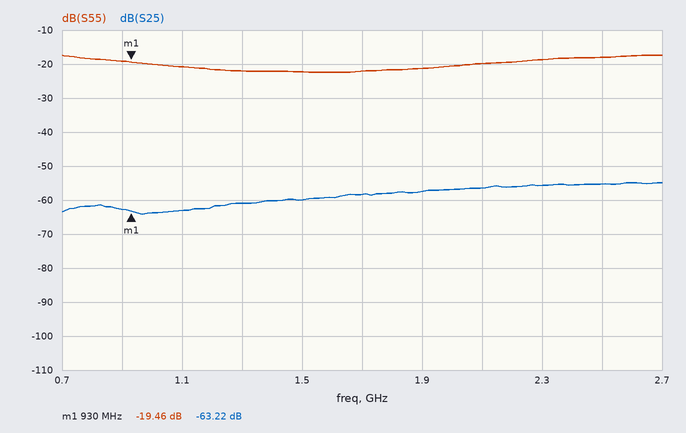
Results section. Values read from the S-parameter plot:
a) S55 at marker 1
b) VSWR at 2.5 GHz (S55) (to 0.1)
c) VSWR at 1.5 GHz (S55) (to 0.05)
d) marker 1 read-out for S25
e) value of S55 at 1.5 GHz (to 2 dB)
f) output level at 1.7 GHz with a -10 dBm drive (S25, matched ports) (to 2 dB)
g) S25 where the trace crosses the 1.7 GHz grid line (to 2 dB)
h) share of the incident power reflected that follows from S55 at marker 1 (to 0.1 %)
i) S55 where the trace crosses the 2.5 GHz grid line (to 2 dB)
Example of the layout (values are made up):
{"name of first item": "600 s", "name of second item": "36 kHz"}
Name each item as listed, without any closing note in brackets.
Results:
{"S55 at marker 1": "-19.46 dB", "VSWR at 2.5 GHz (S55)": "1.3", "VSWR at 1.5 GHz (S55)": "1.15", "marker 1 read-out for S25": "-63.22 dB", "value of S55 at 1.5 GHz": "-22 dB", "output level at 1.7 GHz with a -10 dBm drive (S25, matched ports)": "-68 dBm", "S25 where the trace crosses the 1.7 GHz grid line": "-58 dB", "share of the incident power reflected that follows from S55 at marker 1": "1.1 %", "S55 where the trace crosses the 2.5 GHz grid line": "-18 dB"}
